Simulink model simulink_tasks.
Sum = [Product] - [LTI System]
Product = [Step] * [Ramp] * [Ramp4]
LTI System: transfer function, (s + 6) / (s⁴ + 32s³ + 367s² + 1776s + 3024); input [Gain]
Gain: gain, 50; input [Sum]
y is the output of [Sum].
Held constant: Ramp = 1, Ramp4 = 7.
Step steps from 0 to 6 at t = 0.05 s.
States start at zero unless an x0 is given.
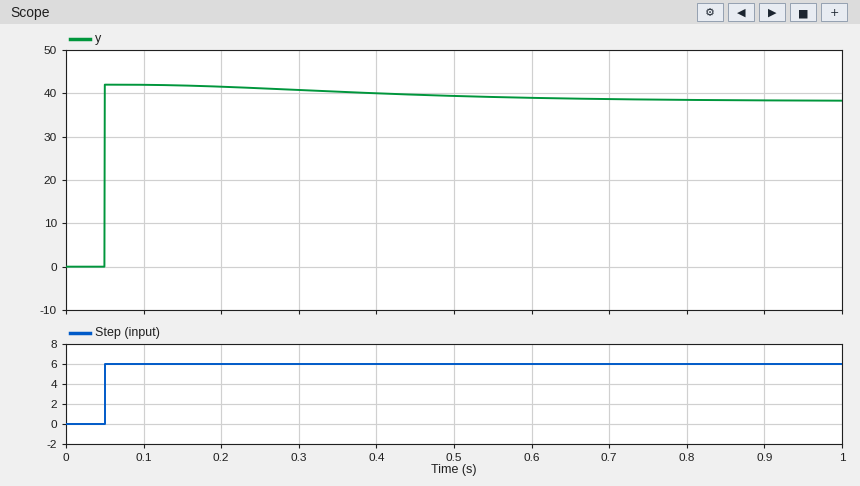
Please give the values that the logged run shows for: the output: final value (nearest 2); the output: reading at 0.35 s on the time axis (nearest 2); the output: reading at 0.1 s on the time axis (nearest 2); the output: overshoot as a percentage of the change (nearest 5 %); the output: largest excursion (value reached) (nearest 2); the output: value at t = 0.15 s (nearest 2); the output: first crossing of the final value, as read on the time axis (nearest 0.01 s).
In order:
38
40
42
10 %
42
42
0.05 s
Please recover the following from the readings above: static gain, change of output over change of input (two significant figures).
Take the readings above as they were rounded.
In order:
6.3
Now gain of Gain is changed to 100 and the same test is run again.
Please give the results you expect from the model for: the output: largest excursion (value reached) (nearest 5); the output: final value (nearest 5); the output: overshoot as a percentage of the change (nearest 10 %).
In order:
40
35
20 %
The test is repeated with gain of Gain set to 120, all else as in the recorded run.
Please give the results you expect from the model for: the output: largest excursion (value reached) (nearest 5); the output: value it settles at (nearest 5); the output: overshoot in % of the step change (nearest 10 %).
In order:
40
35
20 %
